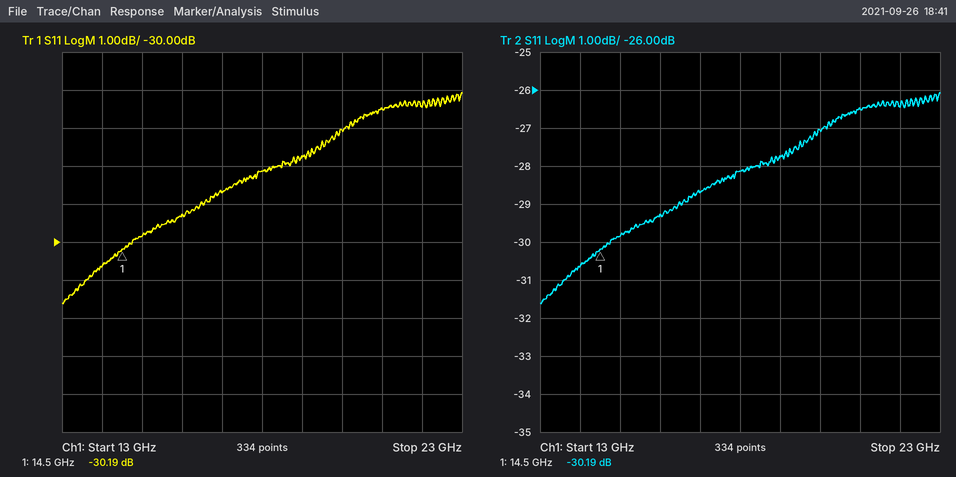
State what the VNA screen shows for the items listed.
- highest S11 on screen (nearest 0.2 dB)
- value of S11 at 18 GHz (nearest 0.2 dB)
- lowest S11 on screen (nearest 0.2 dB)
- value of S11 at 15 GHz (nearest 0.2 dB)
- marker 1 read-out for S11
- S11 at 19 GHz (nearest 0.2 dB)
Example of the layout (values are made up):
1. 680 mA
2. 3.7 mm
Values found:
1. -26.0 dB
2. -28.2 dB
3. -31.6 dB
4. -29.8 dB
5. -30.19 dB
6. -27.8 dB
